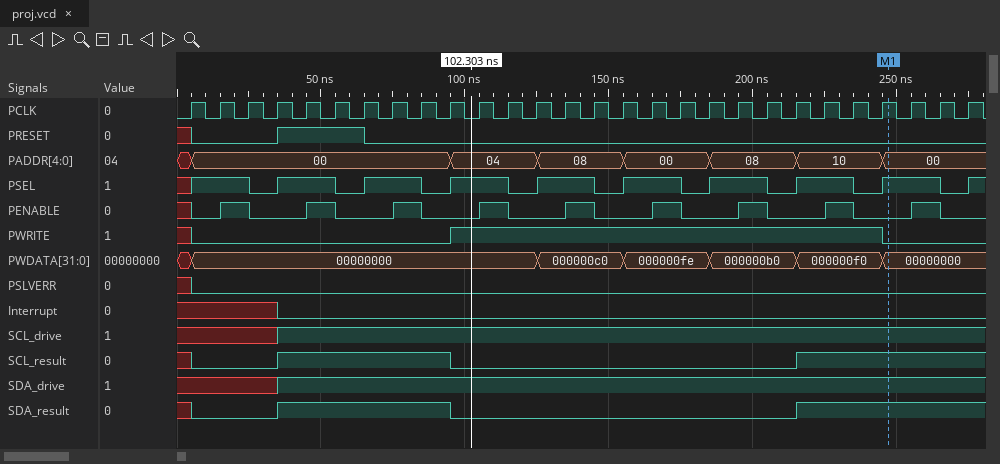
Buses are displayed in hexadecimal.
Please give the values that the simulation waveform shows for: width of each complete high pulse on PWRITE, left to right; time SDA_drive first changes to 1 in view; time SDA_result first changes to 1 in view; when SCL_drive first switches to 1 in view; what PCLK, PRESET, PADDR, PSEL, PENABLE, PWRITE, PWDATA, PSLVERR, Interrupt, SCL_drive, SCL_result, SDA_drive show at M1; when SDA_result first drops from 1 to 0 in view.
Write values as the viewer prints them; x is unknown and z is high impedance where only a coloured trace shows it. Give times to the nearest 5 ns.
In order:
150 ns
35 ns
35 ns
35 ns
PCLK=1, PRESET=0, PADDR=00, PSEL=1, PENABLE=0, PWRITE=0, PWDATA=00000000, PSLVERR=0, Interrupt=0, SCL_drive=1, SCL_result=1, SDA_drive=1
95 ns
